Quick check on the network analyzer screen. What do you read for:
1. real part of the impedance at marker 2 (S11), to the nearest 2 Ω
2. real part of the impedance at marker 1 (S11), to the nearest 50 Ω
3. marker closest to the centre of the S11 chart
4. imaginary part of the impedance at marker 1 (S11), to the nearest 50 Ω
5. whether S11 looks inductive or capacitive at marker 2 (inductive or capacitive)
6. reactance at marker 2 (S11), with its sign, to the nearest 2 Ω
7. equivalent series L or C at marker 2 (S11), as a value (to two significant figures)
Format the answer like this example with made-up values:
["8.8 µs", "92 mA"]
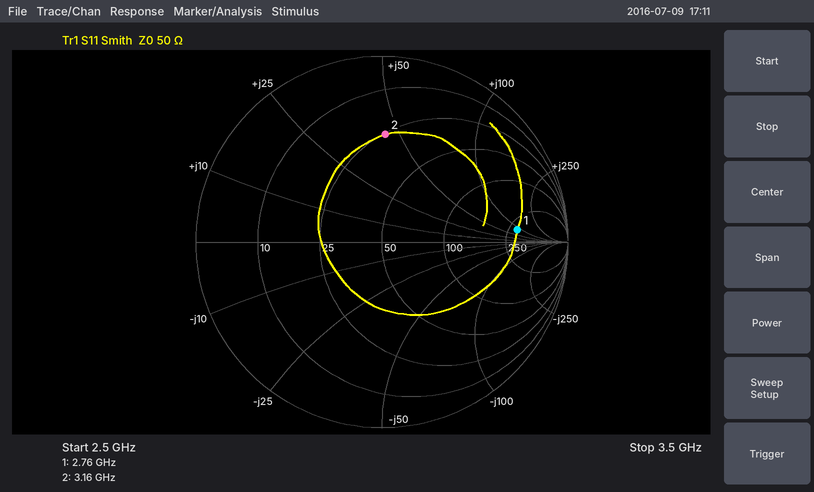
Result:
["26 Ω", "300 Ω", "marker 2", "+100 Ω", "inductive", "+44 Ω", "2.2 nH"]
